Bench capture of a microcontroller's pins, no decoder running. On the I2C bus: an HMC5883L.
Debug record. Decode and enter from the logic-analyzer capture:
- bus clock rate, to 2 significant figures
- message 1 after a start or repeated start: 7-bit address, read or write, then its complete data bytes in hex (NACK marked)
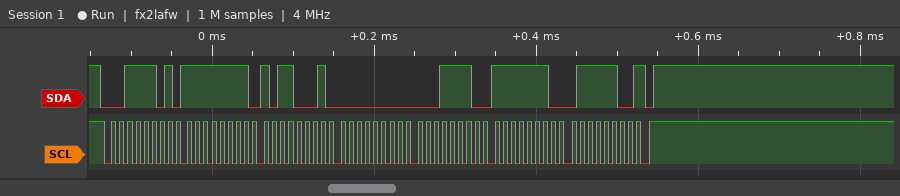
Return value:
100 kHz
0x1E read: FF B1 00 1E FE 7C NACK
